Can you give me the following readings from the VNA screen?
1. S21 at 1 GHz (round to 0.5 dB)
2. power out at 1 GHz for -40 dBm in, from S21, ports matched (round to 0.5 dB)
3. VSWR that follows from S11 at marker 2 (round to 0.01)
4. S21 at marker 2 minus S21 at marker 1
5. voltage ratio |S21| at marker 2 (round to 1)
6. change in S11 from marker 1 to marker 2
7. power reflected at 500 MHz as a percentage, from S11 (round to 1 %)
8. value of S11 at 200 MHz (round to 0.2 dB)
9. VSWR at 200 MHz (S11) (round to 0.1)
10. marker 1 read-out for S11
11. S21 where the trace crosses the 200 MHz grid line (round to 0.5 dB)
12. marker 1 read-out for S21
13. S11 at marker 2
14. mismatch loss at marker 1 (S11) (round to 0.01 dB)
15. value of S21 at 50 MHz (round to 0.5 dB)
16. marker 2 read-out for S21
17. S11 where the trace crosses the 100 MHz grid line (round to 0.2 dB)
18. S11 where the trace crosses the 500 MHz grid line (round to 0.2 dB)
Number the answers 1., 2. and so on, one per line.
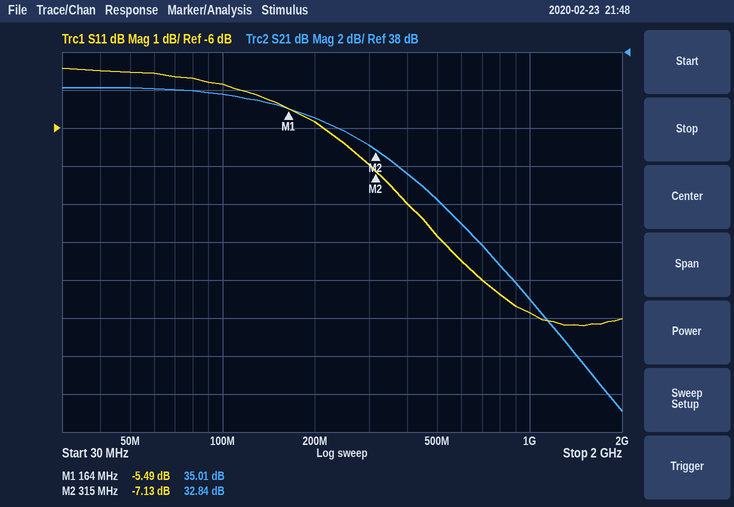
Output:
1. 25.0 dB
2. -15.0 dBm
3. 2.57
4. -2.17 dB
5. 44
6. -1.64 dB
7. 13 %
8. -5.8 dB
9. 3.1
10. -5.49 dB
11. 34.5 dB
12. 35.01 dB
13. -7.13 dB
14. 1.44 dB
15. 36.0 dB
16. 32.84 dB
17. -4.8 dB
18. -8.8 dB
